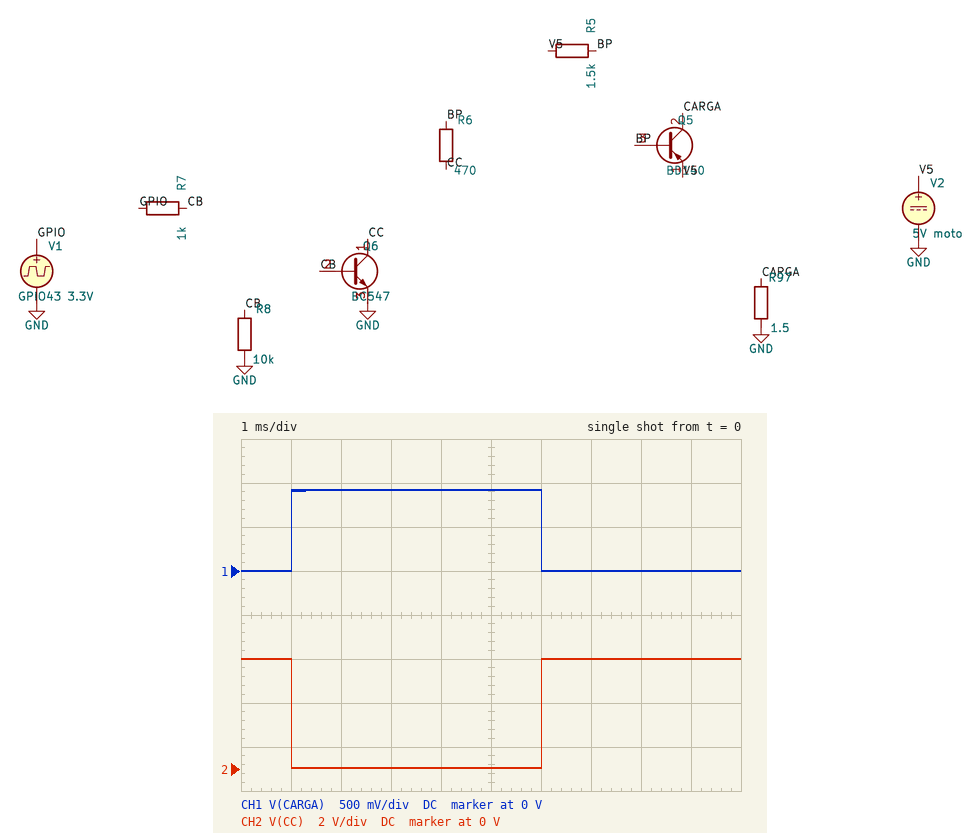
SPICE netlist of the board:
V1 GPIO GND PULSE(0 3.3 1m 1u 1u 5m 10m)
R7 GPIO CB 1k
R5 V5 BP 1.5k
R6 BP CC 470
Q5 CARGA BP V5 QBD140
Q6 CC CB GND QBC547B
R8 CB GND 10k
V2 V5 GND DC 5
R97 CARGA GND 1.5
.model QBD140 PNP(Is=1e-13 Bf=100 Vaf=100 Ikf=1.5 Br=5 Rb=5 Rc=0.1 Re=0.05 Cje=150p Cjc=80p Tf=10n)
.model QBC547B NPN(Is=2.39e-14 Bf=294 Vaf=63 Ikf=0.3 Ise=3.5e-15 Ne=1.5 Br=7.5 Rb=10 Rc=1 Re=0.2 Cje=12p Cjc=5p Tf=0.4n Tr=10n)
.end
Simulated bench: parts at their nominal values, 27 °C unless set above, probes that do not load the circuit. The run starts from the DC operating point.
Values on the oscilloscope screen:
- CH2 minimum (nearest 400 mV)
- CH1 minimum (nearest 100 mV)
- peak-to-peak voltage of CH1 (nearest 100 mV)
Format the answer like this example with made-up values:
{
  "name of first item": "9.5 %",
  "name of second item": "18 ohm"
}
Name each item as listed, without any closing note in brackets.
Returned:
{
  "CH2 minimum": "0 V",
  "CH1 minimum": "0 V",
  "peak-to-peak voltage of CH1": "900 mV"
}
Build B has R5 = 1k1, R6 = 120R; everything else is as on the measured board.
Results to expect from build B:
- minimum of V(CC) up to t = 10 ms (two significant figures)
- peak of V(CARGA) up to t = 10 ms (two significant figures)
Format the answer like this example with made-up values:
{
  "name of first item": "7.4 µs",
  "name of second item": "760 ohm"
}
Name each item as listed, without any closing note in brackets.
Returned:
{
  "minimum of V(CC) up to t = 10 ms": "71 mV",
  "peak of V(CARGA) up to t = 10 ms": "2.4 V"
}
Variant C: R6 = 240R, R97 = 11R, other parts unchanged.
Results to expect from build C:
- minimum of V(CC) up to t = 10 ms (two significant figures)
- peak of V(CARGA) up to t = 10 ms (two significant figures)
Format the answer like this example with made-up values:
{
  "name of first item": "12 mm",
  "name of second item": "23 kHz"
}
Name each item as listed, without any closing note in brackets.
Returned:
{
  "minimum of V(CC) up to t = 10 ms": "42 mV",
  "peak of V(CARGA) up to t = 10 ms": "4.9 V"
}
